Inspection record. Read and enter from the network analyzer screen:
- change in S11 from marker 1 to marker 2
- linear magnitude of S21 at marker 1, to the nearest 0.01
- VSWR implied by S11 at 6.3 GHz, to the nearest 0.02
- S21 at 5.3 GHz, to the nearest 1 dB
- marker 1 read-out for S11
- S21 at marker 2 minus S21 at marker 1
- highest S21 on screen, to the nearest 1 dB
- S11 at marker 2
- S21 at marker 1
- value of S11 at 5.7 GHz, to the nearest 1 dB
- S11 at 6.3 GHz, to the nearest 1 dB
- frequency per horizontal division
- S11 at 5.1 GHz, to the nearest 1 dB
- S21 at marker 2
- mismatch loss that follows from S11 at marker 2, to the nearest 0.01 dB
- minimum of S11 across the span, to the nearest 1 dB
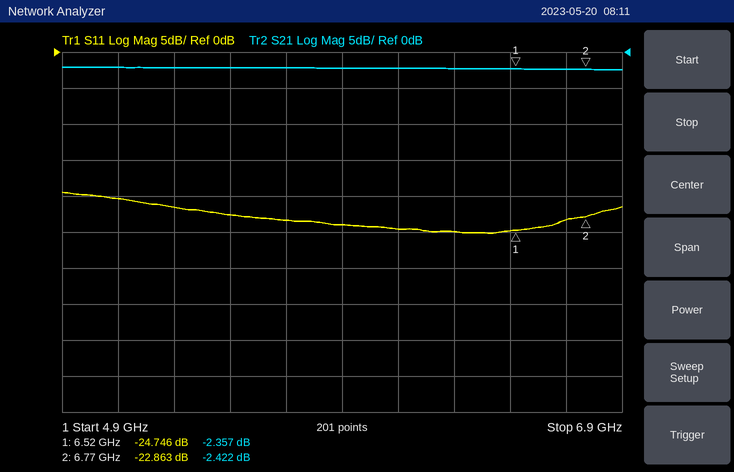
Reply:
1.883 dB
0.76
1.12
-2 dB
-24.746 dB
-0.065 dB
-2 dB
-22.863 dB
-2.357 dB
-23 dB
-25 dB
200 MHz
-20 dB
-2.422 dB
0.02 dB
-25 dB
